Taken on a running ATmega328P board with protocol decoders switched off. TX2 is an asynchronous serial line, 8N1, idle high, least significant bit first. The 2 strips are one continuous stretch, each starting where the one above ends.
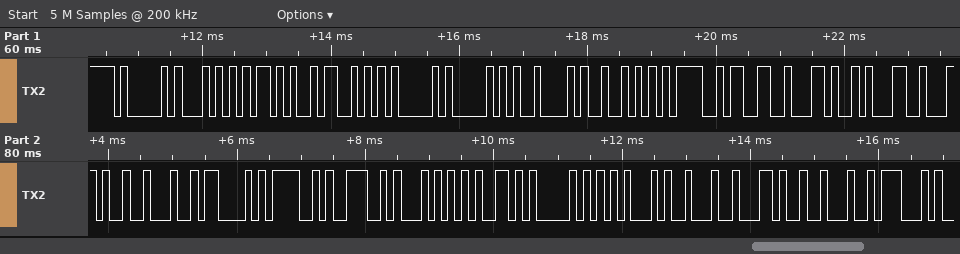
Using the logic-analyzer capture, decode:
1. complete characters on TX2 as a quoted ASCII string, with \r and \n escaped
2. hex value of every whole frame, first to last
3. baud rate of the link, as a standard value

"AT+SAPBR=3,1,\"CONTYPE\",\"G"
41 54 2B 53 41 50 42 52 3D 33 2C 31 2C 22 43 4F 4E 54 59 50 45 22 2C 22 47
9600 baud
